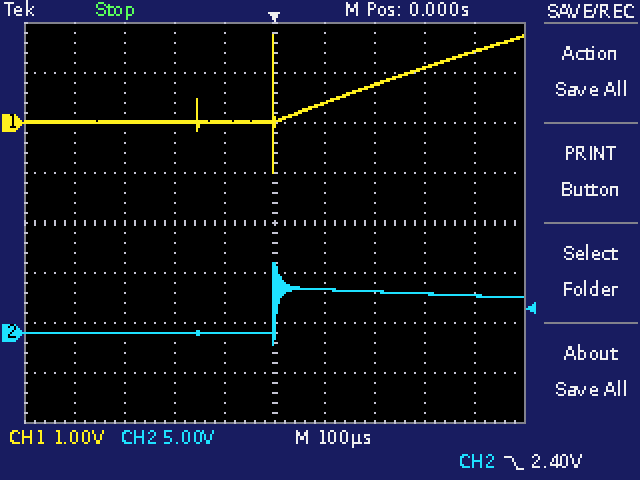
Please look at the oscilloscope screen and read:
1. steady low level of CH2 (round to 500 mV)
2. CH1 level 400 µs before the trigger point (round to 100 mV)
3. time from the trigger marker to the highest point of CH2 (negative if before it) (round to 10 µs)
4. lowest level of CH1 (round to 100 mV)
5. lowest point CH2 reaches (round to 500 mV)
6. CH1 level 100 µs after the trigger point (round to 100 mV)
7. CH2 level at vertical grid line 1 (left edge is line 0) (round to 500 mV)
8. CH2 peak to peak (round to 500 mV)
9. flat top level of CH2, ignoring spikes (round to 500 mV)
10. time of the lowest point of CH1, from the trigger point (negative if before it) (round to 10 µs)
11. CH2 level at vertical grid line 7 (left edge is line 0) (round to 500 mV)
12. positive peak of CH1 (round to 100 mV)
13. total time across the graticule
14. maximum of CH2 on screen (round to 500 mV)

0.0 V
0.0 V
0 µs
-1.0 V
-1.0 V
400 mV
0.0 V
8.0 V
4.0 V
0 µs
4.0 V
1.8 V
1 ms
7.0 V
